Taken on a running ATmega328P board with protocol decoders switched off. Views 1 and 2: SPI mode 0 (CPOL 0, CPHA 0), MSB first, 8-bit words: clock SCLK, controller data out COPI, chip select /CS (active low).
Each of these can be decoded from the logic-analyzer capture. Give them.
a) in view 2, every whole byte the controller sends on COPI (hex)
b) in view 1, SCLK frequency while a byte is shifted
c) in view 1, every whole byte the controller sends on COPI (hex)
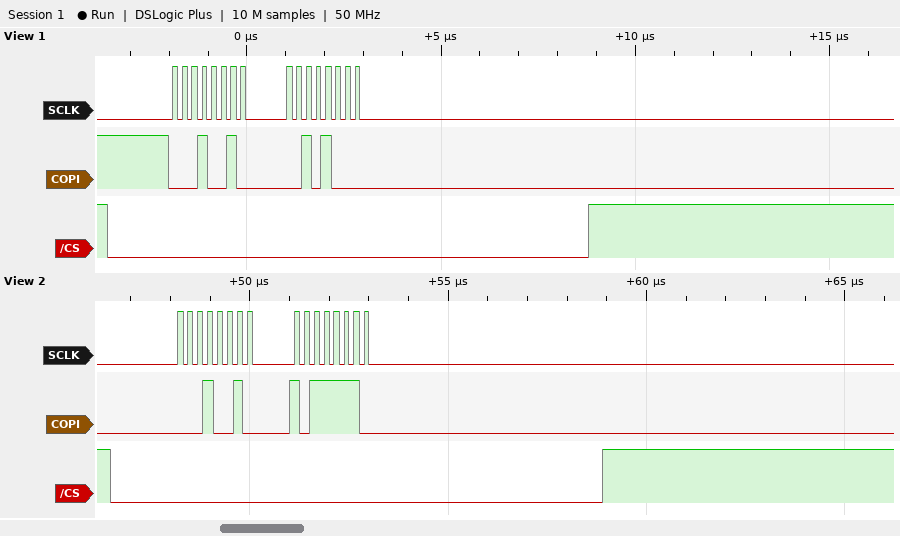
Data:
12 BE
4 MHz
12 28
